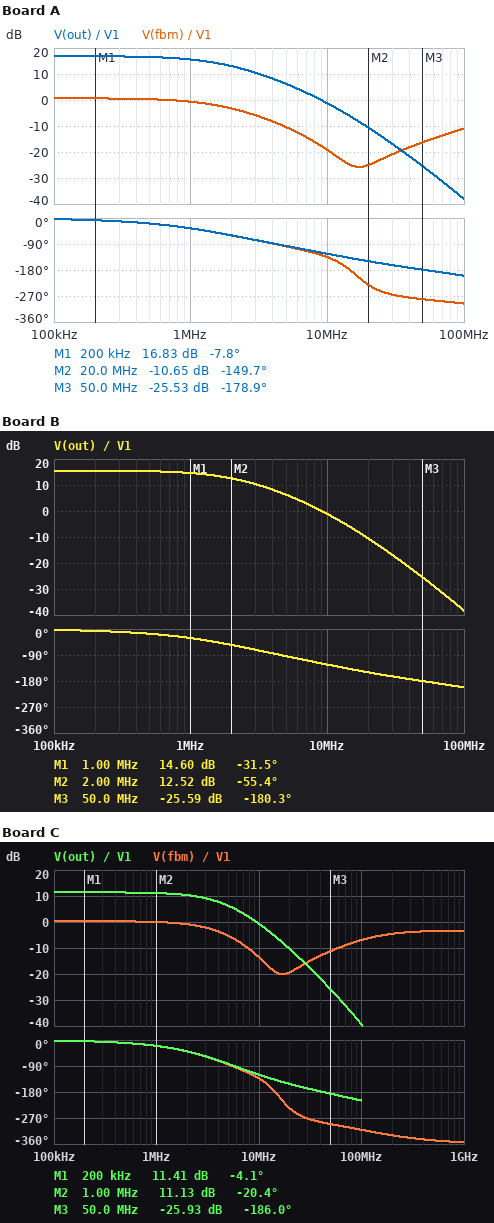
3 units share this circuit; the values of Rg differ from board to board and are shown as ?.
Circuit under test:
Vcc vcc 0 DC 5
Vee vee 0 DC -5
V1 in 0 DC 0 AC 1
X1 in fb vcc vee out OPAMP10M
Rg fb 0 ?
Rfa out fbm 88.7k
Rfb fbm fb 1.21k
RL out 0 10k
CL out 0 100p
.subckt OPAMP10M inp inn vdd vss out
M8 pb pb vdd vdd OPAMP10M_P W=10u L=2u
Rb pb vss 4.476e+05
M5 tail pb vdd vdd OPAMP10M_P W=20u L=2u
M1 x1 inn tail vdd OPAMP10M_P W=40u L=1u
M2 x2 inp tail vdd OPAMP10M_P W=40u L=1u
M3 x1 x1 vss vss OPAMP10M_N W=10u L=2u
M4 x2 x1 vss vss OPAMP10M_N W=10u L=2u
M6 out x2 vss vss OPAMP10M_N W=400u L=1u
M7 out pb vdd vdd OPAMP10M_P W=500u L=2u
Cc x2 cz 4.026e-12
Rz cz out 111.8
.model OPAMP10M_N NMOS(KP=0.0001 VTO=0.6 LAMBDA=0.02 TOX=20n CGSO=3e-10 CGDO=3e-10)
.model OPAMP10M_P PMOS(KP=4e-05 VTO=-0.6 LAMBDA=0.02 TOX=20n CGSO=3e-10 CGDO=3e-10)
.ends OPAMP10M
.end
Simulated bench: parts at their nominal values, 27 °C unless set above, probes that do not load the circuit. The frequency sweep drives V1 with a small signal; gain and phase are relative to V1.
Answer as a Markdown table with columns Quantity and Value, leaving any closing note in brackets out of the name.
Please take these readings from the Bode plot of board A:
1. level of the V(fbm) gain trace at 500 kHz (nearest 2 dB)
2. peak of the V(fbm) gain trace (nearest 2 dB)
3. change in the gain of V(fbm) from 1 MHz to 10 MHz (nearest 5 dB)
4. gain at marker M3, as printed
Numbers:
| Quantity | Value |
|---|---|
| level of the V(fbm) gain trace at 500 kHz | 0 dB |
| peak of the V(fbm) gain trace | 0 dB |
| change in the gain of V(fbm) from 1 MHz to 10 MHz | -20 dB |
| gain at marker M3, as printed | -25.53 dB |
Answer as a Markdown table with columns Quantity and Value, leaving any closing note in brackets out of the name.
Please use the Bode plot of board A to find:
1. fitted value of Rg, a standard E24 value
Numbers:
| Quantity | Value |
|---|---|
| fitted value of Rg, a standard E24 value | 15 kΩ |
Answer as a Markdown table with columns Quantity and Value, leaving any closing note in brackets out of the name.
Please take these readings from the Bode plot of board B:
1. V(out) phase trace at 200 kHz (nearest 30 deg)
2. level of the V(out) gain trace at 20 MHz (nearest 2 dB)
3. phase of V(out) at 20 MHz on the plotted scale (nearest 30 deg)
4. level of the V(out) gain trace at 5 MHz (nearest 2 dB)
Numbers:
| Quantity | Value |
|---|---|
| V(out) phase trace at 200 kHz | 0 deg |
| level of the V(out) gain trace at 20 MHz | -10 dB |
| phase of V(out) at 20 MHz on the plotted scale | -150 deg |
| level of the V(out) gain trace at 5 MHz | 6 dB |
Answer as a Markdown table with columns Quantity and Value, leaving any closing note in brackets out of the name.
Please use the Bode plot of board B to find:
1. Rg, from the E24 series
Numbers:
| Quantity | Value |
|---|---|
| Rg, from the E24 series | 18 kΩ |
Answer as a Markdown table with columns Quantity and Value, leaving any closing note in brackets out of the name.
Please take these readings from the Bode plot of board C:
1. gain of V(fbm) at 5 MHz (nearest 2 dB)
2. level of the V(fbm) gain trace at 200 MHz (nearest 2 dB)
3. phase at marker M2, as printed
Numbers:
| Quantity | Value |
|---|---|
| gain of V(fbm) at 5 MHz | -6 dB |
| level of the V(fbm) gain trace at 200 MHz | -4 dB |
| phase at marker M2, as printed | -20.4 deg |
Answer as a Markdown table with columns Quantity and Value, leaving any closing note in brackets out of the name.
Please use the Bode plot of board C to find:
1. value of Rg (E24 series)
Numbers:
| Quantity | Value |
|---|---|
| value of Rg | 33 kΩ |
